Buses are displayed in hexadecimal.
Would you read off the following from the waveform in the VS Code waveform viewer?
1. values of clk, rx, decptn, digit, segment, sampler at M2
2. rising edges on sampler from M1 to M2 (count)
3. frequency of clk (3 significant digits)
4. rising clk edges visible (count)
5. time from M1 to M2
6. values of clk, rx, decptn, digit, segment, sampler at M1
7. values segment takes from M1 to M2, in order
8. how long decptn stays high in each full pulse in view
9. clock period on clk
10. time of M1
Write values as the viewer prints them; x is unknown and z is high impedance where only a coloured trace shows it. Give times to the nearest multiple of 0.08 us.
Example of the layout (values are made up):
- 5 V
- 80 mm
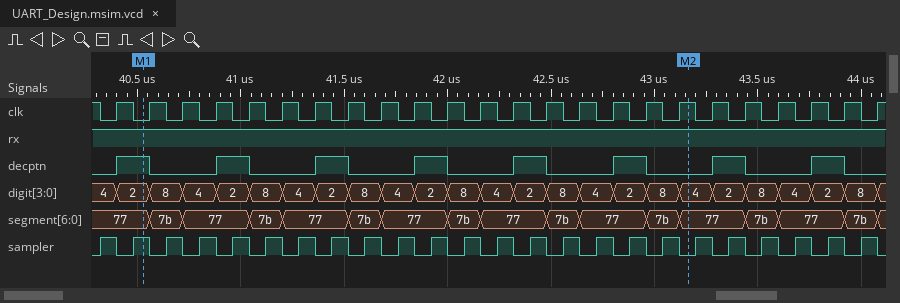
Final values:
- clk=1, rx=1, decptn=0, digit=4, segment=77, sampler=0
- 16
- 6.25 MHz
- 24
- 2.64 us
- clk=0, rx=1, decptn=1, digit=2, segment=77, sampler=1
- 77, 7b, 77, 7b, 77, 7b, 77, 7b, 77, 7b, 77, 7b, 77
- 0.16 us, 0.16 us, 0.16 us, 0.16 us, 0.16 us, 0.16 us, 0.16 us, 0.16 us
- 0.16 us
- 40.56 us
